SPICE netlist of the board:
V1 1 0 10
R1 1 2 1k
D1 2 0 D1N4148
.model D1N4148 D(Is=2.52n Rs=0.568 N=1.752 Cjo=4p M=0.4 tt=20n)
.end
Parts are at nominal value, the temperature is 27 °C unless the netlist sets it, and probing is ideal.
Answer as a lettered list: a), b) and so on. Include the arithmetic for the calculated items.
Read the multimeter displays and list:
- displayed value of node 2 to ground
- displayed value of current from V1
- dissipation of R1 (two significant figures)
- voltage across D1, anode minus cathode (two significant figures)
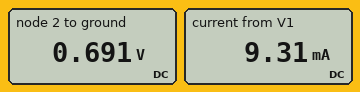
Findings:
a) 0.691 V
b) 9.31 mA
c) (10 V - 691 mV)^2 / 1 kΩ = 87 mW
d) 691 mV = 690 mV
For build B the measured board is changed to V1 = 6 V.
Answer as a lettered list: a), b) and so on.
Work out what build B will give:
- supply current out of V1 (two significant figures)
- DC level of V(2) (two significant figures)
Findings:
a) 5.3 mA
b) 660 mV
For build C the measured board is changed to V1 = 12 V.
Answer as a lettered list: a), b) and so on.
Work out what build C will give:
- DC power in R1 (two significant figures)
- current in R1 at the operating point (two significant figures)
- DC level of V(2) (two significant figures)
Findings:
a) 130 mW
b) 11 mA
c) 700 mV
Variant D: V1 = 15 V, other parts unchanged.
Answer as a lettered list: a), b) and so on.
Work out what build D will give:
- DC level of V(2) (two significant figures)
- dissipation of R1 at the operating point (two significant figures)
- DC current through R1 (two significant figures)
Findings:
a) 710 mV
b) 200 mW
c) 14 mA
